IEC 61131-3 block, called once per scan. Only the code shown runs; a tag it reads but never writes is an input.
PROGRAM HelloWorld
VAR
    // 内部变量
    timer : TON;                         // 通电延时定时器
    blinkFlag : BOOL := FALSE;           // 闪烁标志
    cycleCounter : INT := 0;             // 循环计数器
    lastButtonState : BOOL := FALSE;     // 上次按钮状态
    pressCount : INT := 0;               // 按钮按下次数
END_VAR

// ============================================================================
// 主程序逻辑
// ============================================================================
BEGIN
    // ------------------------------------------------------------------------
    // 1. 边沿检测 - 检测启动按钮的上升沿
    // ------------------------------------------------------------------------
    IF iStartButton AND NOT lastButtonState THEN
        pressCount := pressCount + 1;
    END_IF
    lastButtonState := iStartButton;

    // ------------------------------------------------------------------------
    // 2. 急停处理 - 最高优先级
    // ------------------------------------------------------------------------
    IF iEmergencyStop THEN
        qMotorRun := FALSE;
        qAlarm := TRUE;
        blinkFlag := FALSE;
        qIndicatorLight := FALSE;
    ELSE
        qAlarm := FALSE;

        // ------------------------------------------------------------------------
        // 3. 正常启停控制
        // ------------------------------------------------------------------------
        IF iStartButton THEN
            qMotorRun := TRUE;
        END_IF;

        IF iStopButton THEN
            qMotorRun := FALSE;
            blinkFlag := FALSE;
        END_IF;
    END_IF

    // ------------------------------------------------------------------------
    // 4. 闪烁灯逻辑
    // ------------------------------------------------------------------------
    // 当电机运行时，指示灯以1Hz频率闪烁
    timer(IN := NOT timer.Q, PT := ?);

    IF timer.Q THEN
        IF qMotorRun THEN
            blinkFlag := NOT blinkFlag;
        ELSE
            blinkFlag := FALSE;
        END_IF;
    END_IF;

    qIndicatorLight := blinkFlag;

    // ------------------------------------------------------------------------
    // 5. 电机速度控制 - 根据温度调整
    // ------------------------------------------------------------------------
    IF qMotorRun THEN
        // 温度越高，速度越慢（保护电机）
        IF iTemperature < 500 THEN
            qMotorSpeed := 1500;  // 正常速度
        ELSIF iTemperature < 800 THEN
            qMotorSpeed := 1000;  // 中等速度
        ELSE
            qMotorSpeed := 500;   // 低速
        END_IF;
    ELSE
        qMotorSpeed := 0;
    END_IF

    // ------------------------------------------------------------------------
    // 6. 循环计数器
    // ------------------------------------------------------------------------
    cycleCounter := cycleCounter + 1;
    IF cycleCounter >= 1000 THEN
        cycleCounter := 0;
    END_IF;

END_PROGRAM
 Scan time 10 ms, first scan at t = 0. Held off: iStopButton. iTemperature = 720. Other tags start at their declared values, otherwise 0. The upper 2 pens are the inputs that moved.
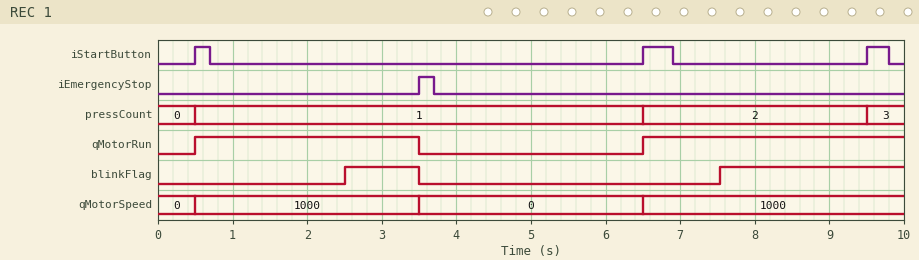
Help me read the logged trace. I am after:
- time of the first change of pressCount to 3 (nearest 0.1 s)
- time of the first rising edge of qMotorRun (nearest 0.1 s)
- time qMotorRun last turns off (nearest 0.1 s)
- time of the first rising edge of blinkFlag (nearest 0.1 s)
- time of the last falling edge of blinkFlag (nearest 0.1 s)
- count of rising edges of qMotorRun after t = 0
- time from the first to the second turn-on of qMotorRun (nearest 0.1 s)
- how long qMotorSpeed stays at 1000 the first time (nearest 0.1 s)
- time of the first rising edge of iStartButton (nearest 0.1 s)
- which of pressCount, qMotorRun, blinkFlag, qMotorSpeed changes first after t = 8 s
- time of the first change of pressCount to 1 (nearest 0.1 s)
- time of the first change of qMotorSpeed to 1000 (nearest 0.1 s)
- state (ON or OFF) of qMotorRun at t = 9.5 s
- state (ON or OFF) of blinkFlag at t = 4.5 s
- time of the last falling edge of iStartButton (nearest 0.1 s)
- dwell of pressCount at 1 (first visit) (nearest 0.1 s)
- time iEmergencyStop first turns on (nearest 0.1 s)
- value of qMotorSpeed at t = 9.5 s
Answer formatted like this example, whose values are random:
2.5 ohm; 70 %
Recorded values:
9.5 s; 0.5 s; 3.5 s; 2.5 s; 3.5 s; 2; 6.0 s; 3.0 s; 0.5 s; pressCount; 0.5 s; 0.5 s; ON; OFF; 9.8 s; 6.0 s; 3.5 s; 1000
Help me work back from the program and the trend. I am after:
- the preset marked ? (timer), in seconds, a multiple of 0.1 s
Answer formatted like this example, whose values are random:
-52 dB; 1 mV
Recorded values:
2.5 s
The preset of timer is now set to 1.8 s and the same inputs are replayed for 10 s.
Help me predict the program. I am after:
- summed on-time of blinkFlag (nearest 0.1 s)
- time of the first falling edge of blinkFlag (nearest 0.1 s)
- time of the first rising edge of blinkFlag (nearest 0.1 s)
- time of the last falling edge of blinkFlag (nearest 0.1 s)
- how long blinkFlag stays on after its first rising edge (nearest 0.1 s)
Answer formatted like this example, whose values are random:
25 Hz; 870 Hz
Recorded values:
3.5 s; 3.5 s; 1.8 s; 9.1 s; 1.7 s
